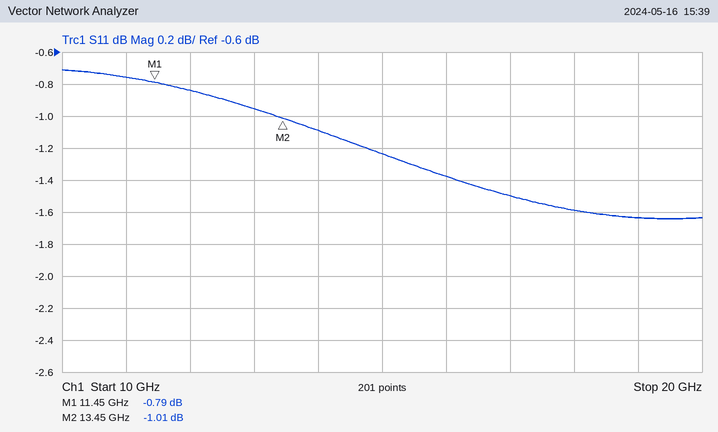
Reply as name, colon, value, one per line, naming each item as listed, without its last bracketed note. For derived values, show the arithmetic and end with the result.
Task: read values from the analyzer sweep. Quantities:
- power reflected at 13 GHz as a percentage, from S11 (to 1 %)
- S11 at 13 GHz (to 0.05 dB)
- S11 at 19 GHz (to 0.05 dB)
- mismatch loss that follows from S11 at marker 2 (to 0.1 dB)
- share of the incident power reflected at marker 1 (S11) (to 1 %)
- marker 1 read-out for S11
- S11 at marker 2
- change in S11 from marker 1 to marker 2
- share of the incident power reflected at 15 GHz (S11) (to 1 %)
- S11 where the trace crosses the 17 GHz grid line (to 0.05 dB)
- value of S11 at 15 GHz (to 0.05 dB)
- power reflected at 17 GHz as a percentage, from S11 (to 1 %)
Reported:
power reflected at 13 GHz as a percentage, from S11: 10^(-0.95/10) ≈ 80 %
S11 at 13 GHz: -0.95 dB
S11 at 19 GHz: -1.65 dB
mismatch loss that follows from S11 at marker 2: −10 log10(1 − 10^(-1.01/10)) ≈ 6.8 dB
share of the incident power reflected at marker 1 (S11): 10^(-0.79/10) ≈ 83 %
marker 1 read-out for S11: -0.79 dB
S11 at marker 2: -1.01 dB
change in S11 from marker 1 to marker 2: -1.01 − (-0.79) = -0.22 dB
share of the incident power reflected at 15 GHz (S11): 10^(-1.25/10) ≈ 75 %
S11 where the trace crosses the 17 GHz grid line: -1.50 dB
value of S11 at 15 GHz: -1.25 dB
power reflected at 17 GHz as a percentage, from S11: 10^(-1.5/10) ≈ 71 %
